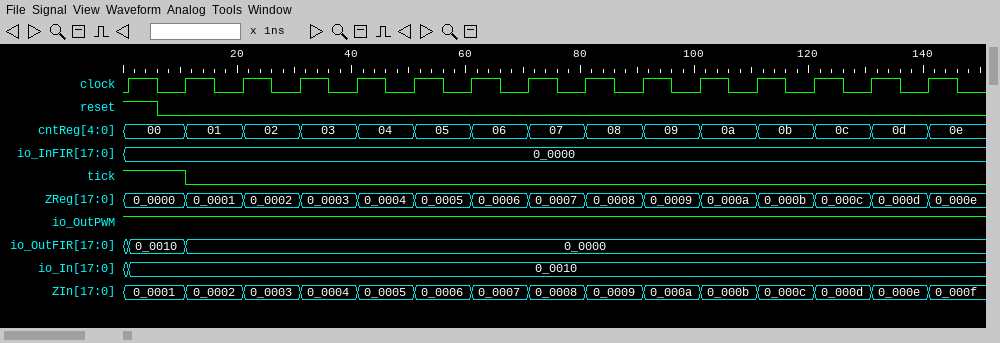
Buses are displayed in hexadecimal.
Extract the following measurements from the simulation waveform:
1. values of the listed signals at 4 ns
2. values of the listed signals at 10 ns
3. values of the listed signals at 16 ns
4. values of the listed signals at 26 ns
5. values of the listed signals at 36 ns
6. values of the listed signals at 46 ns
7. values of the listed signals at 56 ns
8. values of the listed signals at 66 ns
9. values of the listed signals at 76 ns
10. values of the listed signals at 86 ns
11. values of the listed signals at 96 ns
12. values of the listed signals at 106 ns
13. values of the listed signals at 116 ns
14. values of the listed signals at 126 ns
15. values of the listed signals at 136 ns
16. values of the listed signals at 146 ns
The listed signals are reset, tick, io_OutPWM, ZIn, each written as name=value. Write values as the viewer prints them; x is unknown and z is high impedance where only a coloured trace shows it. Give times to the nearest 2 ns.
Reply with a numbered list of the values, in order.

1. reset=1, tick=1, io_OutPWM=1, ZIn=0_0001
2. reset=0, tick=1, io_OutPWM=1, ZIn=0_0001
3. reset=0, tick=0, io_OutPWM=1, ZIn=0_0002
4. reset=0, tick=0, io_OutPWM=1, ZIn=0_0003
5. reset=0, tick=0, io_OutPWM=1, ZIn=0_0004
6. reset=0, tick=0, io_OutPWM=1, ZIn=0_0005
7. reset=0, tick=0, io_OutPWM=1, ZIn=0_0006
8. reset=0, tick=0, io_OutPWM=1, ZIn=0_0007
9. reset=0, tick=0, io_OutPWM=1, ZIn=0_0008
10. reset=0, tick=0, io_OutPWM=1, ZIn=0_0009
11. reset=0, tick=0, io_OutPWM=1, ZIn=0_000a
12. reset=0, tick=0, io_OutPWM=1, ZIn=0_000b
13. reset=0, tick=0, io_OutPWM=1, ZIn=0_000c
14. reset=0, tick=0, io_OutPWM=1, ZIn=0_000d
15. reset=0, tick=0, io_OutPWM=1, ZIn=0_000e
16. reset=0, tick=0, io_OutPWM=1, ZIn=0_000f
